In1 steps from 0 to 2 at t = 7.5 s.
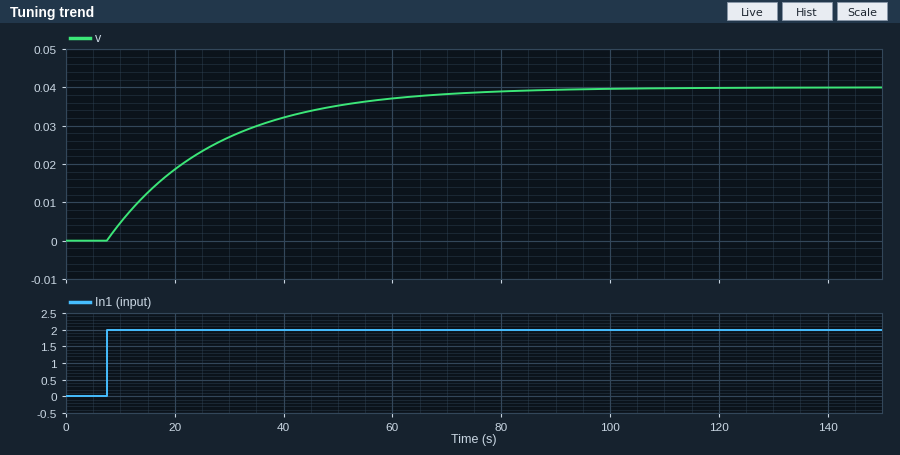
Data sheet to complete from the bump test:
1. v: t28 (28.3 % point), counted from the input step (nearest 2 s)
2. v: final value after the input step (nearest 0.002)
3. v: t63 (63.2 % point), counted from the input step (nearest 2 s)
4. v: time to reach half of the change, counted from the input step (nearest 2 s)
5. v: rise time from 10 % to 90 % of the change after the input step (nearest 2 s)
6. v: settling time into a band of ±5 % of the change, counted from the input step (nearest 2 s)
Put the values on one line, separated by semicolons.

6 s; 0.040; 20 s; 14 s; 44 s; 60 s
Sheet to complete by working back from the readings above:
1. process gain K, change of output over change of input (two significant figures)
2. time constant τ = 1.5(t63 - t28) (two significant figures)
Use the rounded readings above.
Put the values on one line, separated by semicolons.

0.020; 21 s
